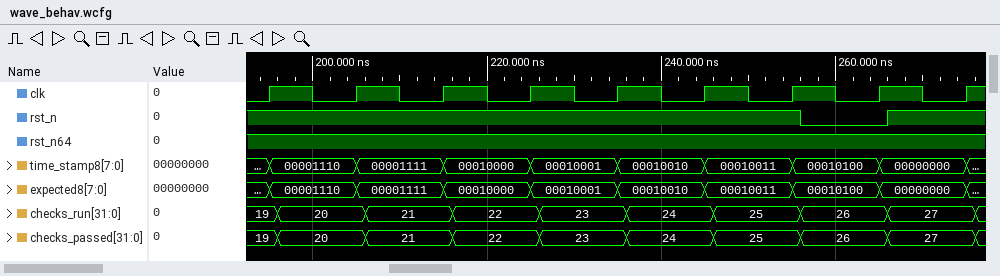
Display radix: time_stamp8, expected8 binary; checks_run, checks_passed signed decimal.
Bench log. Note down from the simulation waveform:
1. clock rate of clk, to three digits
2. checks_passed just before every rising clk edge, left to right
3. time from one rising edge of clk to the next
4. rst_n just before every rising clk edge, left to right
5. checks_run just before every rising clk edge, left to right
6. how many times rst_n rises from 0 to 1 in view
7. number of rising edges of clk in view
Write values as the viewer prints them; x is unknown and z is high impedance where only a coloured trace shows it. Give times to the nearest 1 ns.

100 MHz
19, 20, 21, 22, 23, 24, 25, 26, 27
10 ns
1 1 1 1 1 1 1 0 1
19, 20, 21, 22, 23, 24, 25, 26, 27
1
9
